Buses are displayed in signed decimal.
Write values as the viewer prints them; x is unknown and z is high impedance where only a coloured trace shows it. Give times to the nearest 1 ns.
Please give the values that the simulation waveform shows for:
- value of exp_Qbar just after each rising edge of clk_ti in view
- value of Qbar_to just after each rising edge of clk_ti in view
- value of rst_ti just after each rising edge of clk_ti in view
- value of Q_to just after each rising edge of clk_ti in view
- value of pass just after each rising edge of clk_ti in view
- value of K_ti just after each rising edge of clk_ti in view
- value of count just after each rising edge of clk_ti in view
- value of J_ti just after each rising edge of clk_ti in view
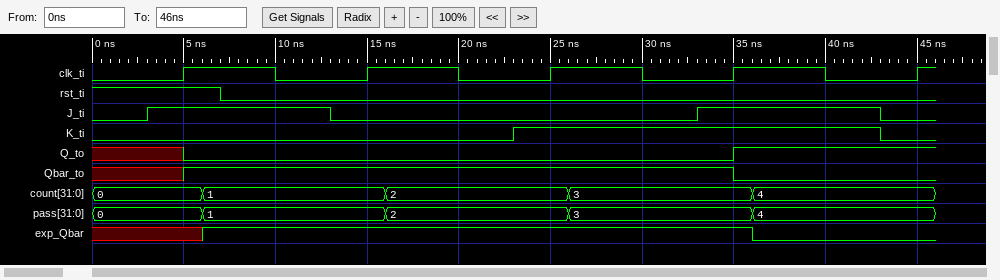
x 1 1 1 0
1 1 1 0 0
1 0 0 0 0
0 0 0 1 1
0, 1, 2, 3, 4
0 0 1 1 0
0, 1, 2, 3, 4
1 0 0 1 0
